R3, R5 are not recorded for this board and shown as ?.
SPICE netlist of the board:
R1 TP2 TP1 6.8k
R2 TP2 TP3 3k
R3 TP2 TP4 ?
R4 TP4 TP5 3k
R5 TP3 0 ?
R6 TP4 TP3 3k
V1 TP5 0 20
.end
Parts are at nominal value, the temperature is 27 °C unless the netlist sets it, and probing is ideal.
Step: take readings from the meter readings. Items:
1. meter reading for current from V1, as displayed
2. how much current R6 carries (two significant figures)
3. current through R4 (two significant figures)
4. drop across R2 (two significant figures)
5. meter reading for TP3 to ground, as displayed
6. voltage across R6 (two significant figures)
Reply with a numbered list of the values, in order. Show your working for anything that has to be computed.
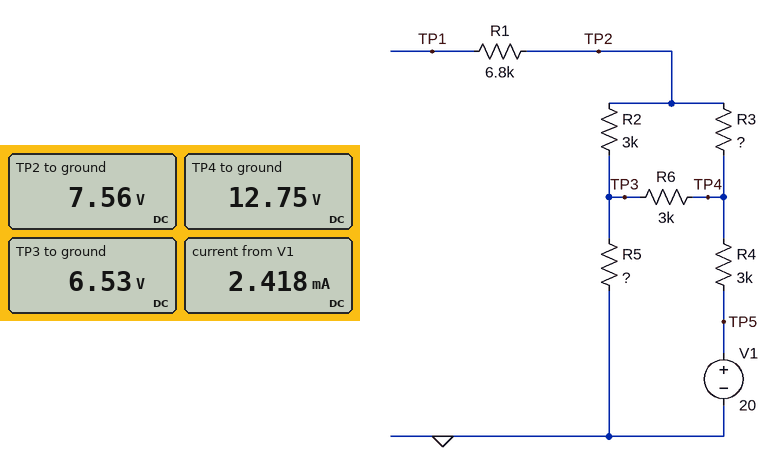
1. 2.418 mA
2. (12.75 V - 6.53 V) / 3 kΩ = 2.1 mA
3. (20 V - 12.75 V) / 3 kΩ = 2.4 mA
4. 7.56 V - 6.53 V = 1.0 V
5. 6.53 V
6. 12.75 V - 6.53 V = 6.2 V
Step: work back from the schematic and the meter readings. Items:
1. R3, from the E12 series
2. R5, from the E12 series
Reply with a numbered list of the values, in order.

1. 15 kΩ
2. 2.7 kΩ
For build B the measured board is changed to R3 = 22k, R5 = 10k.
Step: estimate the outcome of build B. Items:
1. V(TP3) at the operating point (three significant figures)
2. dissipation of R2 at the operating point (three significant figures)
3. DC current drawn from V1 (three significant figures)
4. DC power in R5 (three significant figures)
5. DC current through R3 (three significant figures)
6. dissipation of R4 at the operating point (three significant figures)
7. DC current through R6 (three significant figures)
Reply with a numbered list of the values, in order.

1. 12.8 V
2. 56.0 µW
3. 1.28 mA
4. 16.3 mW
5. 137 µA
6. 4.88 mW
7. 1.14 mA
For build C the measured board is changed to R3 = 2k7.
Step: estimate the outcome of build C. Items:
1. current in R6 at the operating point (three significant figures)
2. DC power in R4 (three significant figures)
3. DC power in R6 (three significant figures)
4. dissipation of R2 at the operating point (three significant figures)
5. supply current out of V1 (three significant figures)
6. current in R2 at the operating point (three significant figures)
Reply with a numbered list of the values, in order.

1. 1.71 mA
2. 20.4 mW
3. 8.77 mW
4. 2.43 mW
5. 2.61 mA
6. 900 µA
